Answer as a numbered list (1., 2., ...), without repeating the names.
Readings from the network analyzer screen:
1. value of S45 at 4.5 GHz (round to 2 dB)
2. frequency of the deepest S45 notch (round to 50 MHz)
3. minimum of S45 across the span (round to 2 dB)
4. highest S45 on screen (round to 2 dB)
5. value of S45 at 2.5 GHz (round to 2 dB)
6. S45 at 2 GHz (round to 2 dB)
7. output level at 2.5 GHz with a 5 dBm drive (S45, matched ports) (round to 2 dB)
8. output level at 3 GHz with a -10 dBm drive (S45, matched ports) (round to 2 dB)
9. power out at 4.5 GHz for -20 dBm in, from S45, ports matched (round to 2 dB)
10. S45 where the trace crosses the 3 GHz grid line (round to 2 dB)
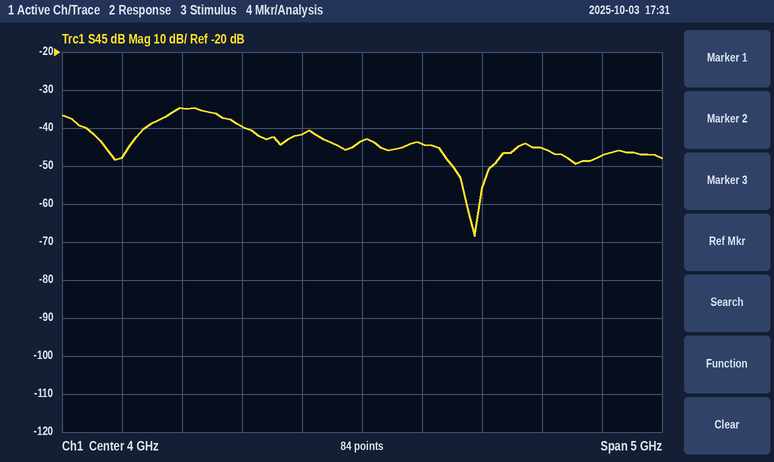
1. -44 dB
2. 4.95 GHz
3. -68 dB
4. -34 dB
5. -34 dB
6. -48 dB
7. -30 dBm
8. -50 dBm
9. -64 dBm
10. -40 dB
